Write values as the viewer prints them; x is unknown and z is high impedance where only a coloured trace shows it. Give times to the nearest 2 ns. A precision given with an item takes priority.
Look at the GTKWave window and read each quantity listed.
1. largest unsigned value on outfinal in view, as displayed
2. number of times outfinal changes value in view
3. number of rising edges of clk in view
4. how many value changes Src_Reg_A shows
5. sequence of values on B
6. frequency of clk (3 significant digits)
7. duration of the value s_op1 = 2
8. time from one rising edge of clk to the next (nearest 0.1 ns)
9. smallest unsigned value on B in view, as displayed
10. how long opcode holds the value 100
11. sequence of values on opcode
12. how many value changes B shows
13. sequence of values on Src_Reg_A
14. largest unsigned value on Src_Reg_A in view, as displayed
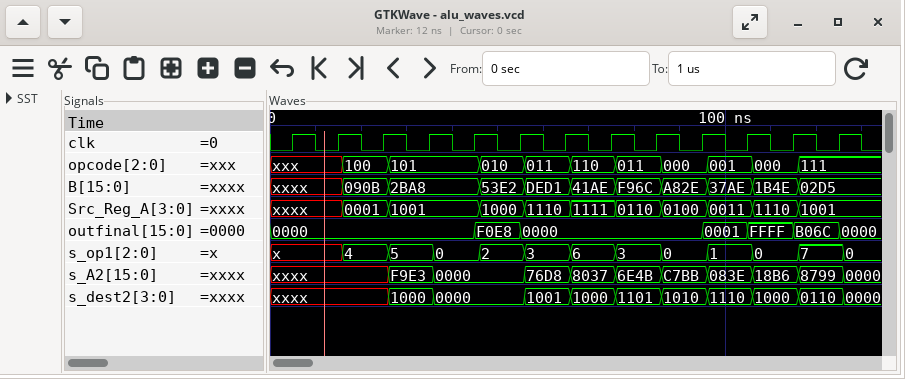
FFFF
6
13
10
xxxx, 090B, 2BA8, 53E2, DED1, 41AE, F96C, A82E, 37AE, 1B4E, 02D5
100 MHz
10 ns
10 ns
02D5
10 ns
xxx, 100, 101, 010, 011, 110, 011, 000, 001, 000, 111
10
xxxx, 0001, 1001, 1000, 1110, 1111, 0110, 0100, 0011, 1110, 1001
1111
